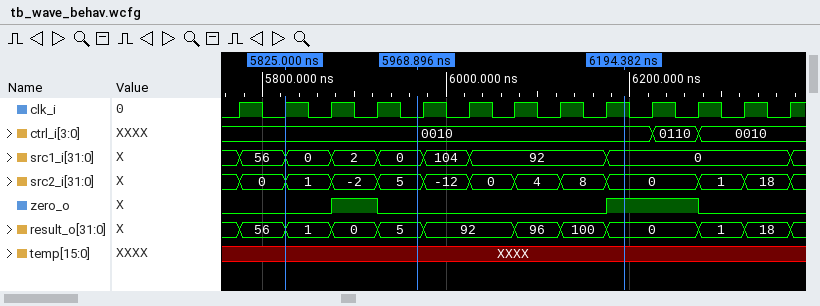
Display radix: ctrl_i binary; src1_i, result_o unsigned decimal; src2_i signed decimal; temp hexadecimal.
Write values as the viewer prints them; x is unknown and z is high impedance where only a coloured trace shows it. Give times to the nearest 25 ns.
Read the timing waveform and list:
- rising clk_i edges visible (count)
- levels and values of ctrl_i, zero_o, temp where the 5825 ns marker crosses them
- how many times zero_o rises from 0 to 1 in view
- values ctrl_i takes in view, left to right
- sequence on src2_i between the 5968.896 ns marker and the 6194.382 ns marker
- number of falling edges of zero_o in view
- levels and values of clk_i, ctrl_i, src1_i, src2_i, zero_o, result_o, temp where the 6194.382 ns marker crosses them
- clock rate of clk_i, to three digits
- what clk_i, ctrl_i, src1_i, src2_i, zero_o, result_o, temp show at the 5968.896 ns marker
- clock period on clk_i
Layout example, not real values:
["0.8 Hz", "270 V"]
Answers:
["13", "ctrl_i=0010, zero_o=0, temp=XXXX", "2", "0010, 0110, 0010", "5, -12, 0, 4, 8, 0", "2", "clk_i=1, ctrl_i=0010, src1_i=0, src2_i=0, zero_o=1, result_o=0, temp=XXXX", "20.0 MHz", "clk_i=0, ctrl_i=0010, src1_i=0, src2_i=5, zero_o=0, result_o=5, temp=XXXX", "50 ns"]
